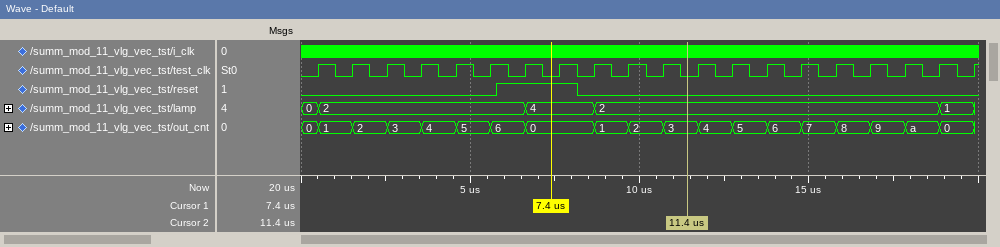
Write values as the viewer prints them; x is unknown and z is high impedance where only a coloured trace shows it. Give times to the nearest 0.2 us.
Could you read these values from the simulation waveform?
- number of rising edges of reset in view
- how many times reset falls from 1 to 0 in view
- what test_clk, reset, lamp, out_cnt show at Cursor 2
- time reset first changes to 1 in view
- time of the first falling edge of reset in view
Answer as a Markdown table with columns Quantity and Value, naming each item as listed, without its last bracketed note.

| Quantity | Value |
|---|---|
| number of rising edges of reset in view | 1 |
| how many times reset falls from 1 to 0 in view | 1 |
| what test_clk, reset, lamp, out_cnt show at Cursor 2 | test_clk=0, reset=0, lamp=2, out_cnt=3 |
| time reset first changes to 1 in view | 5.8 us |
| time of the first falling edge of reset in view | 8.2 us |
